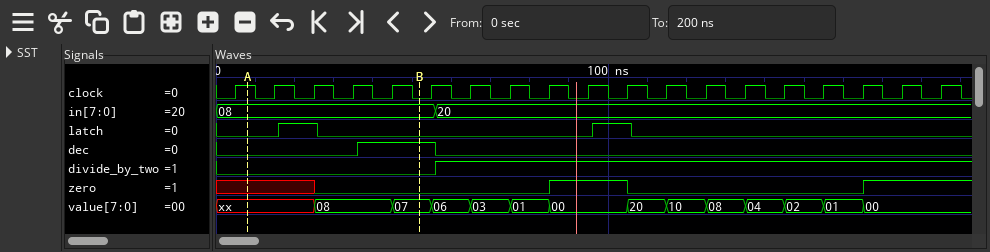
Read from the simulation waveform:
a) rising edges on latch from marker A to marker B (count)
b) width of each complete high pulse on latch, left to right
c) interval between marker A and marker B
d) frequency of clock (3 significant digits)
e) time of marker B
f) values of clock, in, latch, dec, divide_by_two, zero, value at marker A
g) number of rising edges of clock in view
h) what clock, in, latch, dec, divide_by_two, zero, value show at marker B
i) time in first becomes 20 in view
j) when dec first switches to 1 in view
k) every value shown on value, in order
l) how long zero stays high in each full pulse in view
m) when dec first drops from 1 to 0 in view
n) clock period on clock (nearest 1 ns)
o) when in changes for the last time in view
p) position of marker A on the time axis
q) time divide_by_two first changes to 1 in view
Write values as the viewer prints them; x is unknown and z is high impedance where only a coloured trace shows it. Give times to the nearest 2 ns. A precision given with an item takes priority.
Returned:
1
10 ns, 10 ns
44 ns
100 MHz
52 ns
clock=1, in=08, latch=0, dec=0, divide_by_two=0, zero=x, value=xx
19
clock=0, in=08, latch=0, dec=1, divide_by_two=0, zero=0, value=07
56 ns
36 ns
xx, 08, 07, 06, 03, 01, 00, 20, 10, 08, 04, 02, 01, 00
20 ns
56 ns
10 ns
56 ns
8 ns
56 ns
